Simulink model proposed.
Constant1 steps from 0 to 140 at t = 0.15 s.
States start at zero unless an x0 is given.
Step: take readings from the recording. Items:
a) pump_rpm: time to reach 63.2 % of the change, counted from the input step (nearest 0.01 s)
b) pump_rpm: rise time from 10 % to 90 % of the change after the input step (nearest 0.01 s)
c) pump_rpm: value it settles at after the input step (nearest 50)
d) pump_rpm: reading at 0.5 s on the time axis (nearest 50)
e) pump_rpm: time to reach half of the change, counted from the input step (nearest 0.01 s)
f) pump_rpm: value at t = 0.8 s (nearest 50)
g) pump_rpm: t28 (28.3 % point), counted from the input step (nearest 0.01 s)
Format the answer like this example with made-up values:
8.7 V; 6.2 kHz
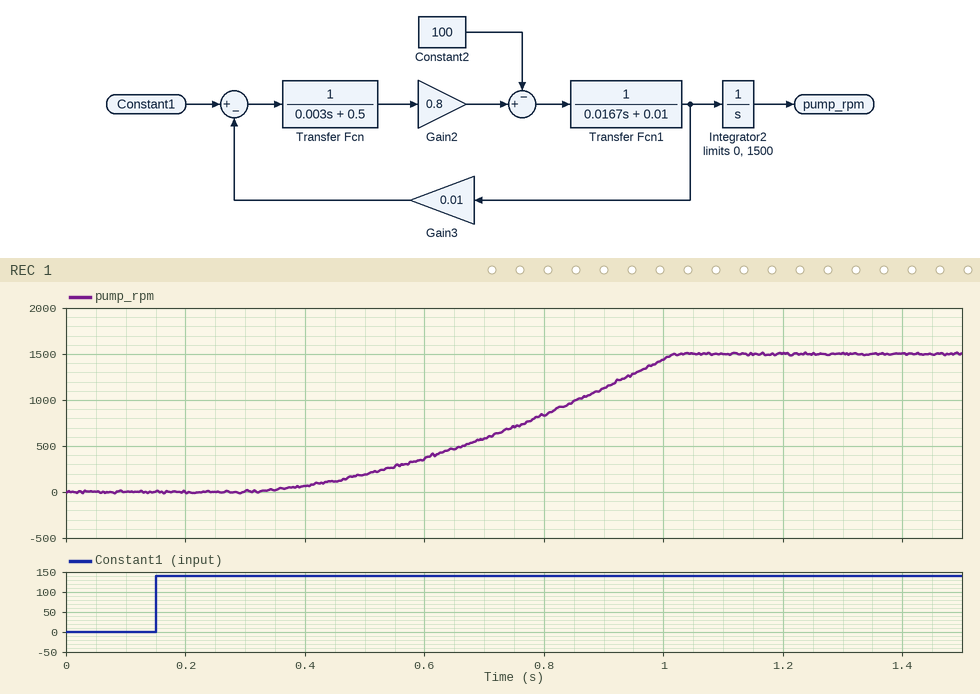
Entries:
0.69 s; 0.50 s; 1500; 200; 0.62 s; 850; 0.48 s
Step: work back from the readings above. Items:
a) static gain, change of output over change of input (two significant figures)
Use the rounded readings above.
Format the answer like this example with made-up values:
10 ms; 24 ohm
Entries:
11
